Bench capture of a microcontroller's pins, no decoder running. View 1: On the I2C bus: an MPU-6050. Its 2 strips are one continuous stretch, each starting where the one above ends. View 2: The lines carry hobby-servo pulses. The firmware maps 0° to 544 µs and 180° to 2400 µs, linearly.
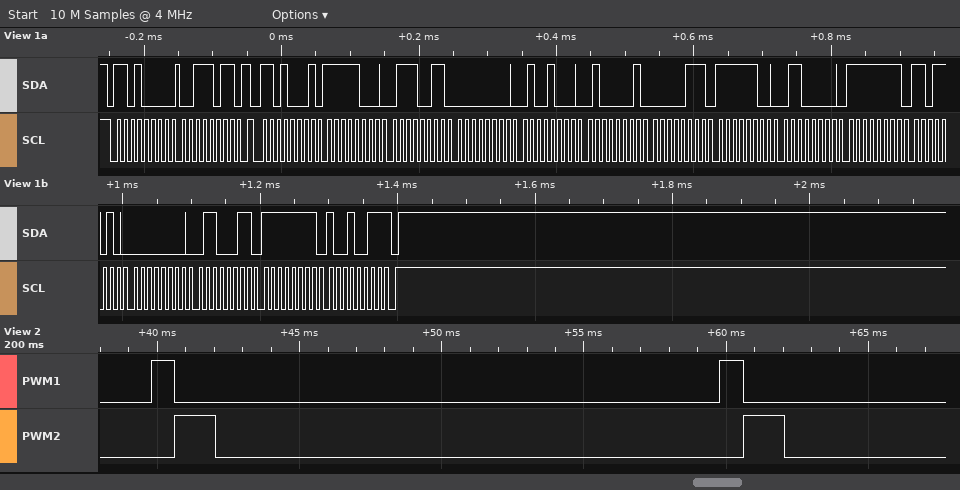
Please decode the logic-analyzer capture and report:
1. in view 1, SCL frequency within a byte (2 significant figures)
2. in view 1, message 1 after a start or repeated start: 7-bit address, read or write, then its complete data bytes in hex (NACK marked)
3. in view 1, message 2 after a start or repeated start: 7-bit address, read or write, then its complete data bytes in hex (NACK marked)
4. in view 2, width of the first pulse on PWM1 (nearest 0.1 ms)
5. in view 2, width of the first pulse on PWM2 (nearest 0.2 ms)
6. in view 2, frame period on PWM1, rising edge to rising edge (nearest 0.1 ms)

100 kHz
0x68 write: 3B
0x68 read: F8 73 00 48 41 07 FC 60 FF DA 00 63 FF 93 NACK
0.8 ms
1.4 ms
20.0 ms
